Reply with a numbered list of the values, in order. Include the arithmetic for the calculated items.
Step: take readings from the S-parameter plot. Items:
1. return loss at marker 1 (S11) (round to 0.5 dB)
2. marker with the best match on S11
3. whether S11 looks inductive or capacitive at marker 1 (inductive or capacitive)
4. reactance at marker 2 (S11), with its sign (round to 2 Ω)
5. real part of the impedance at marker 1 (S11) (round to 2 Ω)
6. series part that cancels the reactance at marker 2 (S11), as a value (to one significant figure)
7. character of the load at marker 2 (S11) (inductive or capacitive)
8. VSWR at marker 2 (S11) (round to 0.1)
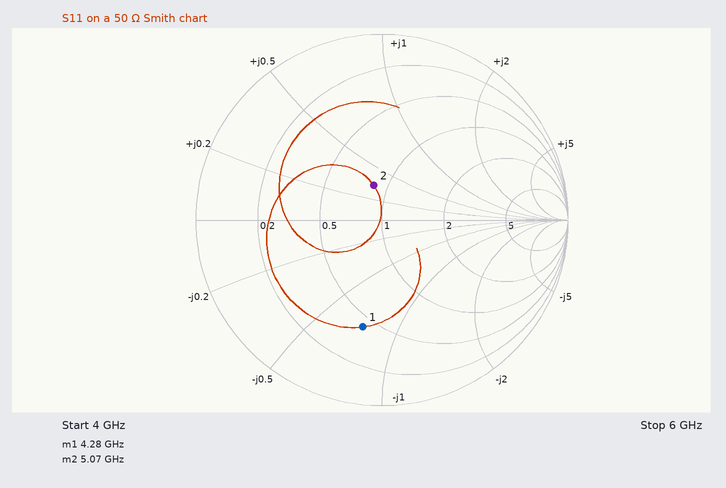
1. 4.5 dB
2. marker 2
3. capacitive
4. +16 Ω
5. 22 Ω
6. C = 1/(2π × 5.07 GHz × 16 Ω) ≈ 2 pF
7. inductive
8. 1.5
